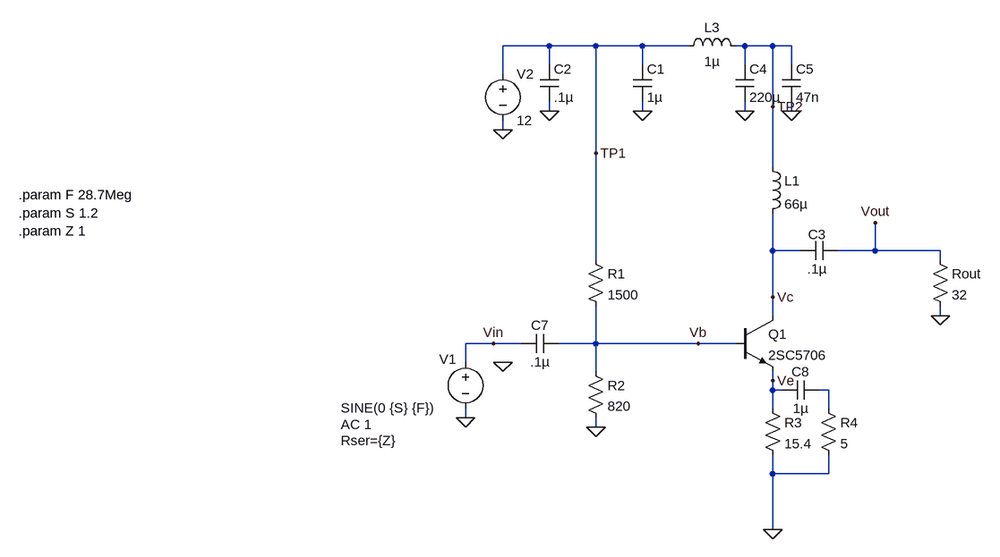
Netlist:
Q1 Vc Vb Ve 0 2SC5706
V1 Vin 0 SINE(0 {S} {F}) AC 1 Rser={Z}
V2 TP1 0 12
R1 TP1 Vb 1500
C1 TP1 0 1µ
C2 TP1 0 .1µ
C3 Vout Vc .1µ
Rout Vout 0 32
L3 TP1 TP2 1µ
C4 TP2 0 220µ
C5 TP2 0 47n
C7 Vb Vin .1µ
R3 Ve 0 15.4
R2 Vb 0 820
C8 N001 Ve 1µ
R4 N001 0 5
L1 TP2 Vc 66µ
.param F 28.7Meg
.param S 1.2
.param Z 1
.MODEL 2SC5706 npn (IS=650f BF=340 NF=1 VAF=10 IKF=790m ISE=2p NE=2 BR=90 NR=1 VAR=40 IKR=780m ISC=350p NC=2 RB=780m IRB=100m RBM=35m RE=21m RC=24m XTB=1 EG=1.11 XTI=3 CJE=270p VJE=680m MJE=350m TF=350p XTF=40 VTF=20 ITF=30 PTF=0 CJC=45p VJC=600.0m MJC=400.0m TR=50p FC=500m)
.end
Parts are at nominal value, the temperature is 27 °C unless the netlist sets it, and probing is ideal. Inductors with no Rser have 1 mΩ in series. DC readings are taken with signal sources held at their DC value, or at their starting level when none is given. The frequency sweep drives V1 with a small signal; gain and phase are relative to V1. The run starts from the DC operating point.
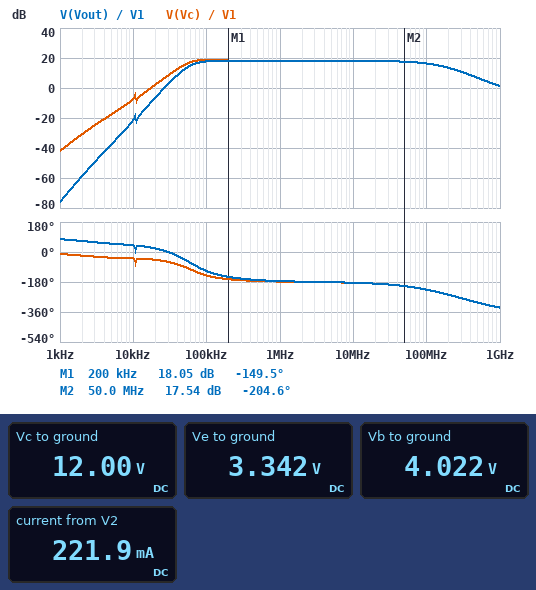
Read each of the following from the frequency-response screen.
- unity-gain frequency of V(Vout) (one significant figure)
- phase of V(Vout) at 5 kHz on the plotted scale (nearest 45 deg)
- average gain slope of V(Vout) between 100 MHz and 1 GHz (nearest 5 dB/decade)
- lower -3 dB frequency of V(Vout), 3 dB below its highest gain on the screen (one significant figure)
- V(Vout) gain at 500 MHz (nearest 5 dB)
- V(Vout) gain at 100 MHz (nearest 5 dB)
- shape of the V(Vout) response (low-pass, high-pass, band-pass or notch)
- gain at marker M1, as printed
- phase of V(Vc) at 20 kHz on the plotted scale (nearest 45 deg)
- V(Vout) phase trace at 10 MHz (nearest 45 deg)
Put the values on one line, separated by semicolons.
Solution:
30 kHz; 45 deg; -15 dB/decade; 60 kHz; 5 dB; 15 dB; band-pass; 18.05 dB; -45 deg; -180 deg
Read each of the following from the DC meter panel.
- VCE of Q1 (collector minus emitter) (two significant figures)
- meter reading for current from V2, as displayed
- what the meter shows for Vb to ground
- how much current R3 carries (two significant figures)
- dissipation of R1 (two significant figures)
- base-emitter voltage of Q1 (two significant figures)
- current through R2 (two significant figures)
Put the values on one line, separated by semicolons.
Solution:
8.7 V; 221.9 mA; 4.022 V; 220 mA; 42 mW; 680 mV; 4.9 mA
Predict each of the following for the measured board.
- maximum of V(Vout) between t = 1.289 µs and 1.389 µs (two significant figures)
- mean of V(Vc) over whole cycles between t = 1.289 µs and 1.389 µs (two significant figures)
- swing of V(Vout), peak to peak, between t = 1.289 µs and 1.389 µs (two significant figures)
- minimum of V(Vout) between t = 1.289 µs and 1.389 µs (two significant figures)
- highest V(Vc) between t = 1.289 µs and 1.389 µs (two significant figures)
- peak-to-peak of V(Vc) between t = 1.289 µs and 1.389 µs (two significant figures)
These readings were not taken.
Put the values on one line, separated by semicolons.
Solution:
7.1 V; 12 V; 15 V; -7.8 V; 19 V; 15 V
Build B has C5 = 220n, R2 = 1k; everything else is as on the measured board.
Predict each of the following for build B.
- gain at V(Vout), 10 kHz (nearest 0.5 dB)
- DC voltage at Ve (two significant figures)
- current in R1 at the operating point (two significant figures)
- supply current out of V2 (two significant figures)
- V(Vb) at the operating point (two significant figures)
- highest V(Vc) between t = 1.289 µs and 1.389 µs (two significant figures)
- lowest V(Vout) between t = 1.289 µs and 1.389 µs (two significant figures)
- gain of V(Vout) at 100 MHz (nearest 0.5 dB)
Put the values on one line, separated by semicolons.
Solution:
-21.0 dB; 3.8 V; 5.0 mA; 250 mA; 4.5 V; 20 V; -7.5 V; 16.5 dB
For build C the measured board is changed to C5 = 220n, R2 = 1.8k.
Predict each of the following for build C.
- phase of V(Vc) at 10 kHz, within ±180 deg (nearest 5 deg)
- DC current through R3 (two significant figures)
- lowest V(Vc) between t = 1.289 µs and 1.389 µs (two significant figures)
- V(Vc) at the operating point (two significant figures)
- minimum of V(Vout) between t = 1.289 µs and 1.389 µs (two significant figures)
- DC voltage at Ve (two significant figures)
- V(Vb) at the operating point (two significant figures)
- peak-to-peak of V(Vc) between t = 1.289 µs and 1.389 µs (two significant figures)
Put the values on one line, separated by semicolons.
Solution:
-45 deg; 340 mA; 5.5 V; 12 V; -6.6 V; 5.2 V; 5.9 V; 16 V
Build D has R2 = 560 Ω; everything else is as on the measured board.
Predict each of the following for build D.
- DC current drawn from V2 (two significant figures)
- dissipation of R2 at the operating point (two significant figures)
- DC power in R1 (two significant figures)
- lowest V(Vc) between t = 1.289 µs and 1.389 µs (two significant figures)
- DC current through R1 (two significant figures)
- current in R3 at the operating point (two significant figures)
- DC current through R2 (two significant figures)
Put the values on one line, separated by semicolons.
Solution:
170 mA; 18 mW; 52 mW; 3.6 V; 5.9 mA; 160 mA; 5.6 mA
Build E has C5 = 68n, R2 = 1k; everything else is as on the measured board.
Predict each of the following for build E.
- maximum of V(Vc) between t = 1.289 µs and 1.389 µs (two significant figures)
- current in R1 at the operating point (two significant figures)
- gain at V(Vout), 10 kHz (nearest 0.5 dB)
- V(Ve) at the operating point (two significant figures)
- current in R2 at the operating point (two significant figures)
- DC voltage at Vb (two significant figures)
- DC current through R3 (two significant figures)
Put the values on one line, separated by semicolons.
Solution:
20 V; 5.0 mA; -21.0 dB; 3.8 V; 4.5 mA; 4.5 V; 250 mA
